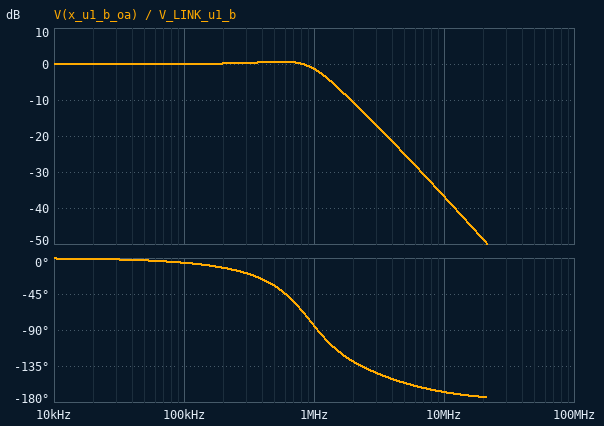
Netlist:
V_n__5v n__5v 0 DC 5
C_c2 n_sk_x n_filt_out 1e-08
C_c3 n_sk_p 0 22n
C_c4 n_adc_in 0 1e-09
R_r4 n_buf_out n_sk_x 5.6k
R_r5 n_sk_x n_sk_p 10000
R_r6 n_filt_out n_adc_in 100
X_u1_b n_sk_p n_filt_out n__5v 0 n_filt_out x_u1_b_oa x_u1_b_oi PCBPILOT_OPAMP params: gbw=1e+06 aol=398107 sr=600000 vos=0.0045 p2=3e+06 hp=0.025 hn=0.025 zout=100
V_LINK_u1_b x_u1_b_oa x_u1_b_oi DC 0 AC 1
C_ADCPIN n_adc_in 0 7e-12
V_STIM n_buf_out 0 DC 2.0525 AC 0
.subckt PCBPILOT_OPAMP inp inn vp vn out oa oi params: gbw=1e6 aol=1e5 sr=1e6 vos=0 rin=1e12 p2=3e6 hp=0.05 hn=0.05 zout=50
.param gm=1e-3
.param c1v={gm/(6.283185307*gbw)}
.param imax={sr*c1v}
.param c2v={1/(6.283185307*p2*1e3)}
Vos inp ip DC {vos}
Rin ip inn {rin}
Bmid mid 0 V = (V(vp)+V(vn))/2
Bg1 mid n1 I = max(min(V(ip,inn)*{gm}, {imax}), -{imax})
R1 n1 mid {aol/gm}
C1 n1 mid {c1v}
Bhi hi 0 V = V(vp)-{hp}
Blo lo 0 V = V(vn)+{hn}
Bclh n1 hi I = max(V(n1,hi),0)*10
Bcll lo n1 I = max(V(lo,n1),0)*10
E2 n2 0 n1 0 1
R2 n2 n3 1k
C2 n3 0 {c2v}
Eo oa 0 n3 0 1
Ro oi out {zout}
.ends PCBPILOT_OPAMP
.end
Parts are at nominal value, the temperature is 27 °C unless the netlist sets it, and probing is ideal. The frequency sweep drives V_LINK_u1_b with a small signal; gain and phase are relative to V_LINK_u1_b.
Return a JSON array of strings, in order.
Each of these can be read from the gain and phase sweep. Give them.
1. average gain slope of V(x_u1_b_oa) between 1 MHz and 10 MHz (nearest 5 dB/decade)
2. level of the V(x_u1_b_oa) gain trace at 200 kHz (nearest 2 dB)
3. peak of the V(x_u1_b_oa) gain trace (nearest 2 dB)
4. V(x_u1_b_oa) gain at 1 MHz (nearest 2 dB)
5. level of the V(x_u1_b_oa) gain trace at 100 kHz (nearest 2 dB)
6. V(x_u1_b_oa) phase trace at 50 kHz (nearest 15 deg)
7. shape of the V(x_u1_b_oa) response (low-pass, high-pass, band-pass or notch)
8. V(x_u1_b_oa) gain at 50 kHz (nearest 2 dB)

["-35 dB/decade", "0 dB", "0 dB", "-2 dB", "0 dB", "0 deg", "low-pass", "0 dB"]
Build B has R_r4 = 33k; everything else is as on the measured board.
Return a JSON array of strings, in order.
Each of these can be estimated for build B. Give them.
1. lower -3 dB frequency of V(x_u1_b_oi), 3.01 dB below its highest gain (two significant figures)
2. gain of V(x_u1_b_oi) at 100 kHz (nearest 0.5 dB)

["690 kHz", "-20.0 dB"]
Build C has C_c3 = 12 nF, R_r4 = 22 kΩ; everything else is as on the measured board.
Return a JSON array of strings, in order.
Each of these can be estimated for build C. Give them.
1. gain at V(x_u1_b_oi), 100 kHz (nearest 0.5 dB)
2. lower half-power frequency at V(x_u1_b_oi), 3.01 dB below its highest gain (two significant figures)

["-20.0 dB", "690 kHz"]
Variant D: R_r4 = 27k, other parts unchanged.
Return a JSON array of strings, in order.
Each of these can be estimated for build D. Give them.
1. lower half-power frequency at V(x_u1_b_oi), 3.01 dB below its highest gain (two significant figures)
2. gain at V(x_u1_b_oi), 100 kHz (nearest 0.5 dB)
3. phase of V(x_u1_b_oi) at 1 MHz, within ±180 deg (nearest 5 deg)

["690 kHz", "-20.0 dB", "-135 deg"]
